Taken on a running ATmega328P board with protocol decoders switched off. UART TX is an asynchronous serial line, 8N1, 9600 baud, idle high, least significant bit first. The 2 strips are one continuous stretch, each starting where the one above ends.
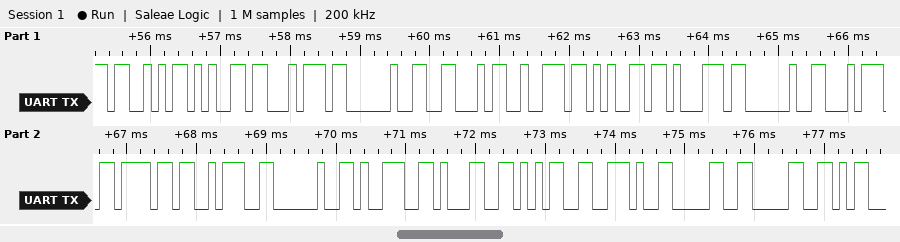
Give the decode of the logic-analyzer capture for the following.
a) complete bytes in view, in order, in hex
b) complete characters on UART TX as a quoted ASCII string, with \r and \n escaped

53 65 74 20 46 72 65 71 20 74 6F 3A 20 39 31 35 2E 30 30
"Set Freq to: 915.00"
